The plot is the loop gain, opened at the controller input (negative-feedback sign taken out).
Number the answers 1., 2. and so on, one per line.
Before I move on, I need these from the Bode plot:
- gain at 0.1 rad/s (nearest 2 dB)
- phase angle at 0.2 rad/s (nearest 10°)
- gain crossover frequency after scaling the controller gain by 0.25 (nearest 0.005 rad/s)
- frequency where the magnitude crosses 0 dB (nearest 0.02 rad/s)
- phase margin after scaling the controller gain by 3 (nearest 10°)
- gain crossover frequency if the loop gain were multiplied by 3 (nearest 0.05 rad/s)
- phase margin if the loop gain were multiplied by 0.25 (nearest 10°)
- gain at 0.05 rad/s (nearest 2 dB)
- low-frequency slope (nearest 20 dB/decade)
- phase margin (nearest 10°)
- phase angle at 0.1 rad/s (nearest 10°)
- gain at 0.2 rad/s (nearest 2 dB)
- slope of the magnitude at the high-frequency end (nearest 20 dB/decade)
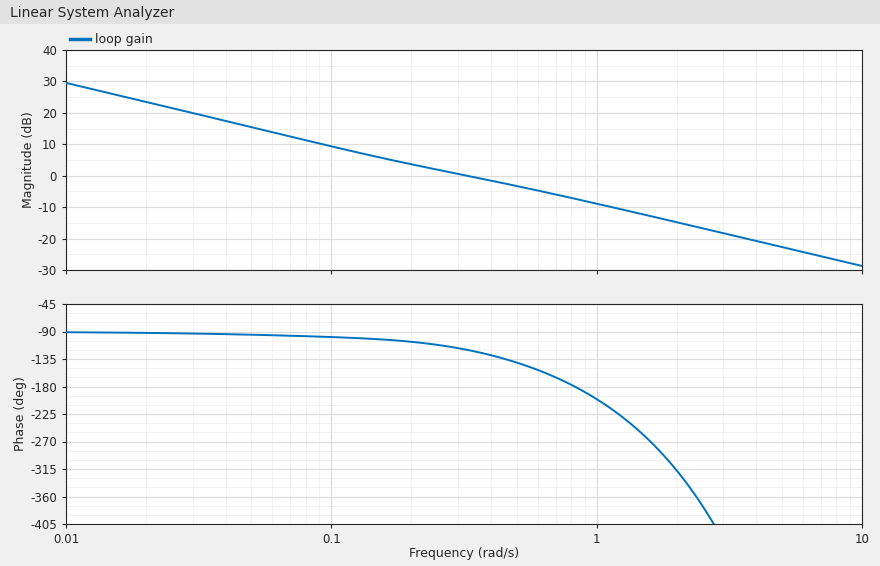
1. 10 dB
2. -110°
3. 0.075 rad/s
4. 0.32 rad/s
5. -30°
6. 1.10 rad/s
7. 80°
8. 16 dB
9. -20 dB/decade
10. 60°
11. -100°
12. 4 dB
13. -20 dB/decade
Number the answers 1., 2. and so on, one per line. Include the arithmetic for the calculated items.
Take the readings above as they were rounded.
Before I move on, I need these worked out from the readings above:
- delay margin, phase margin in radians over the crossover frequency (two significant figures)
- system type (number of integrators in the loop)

1. 60 × π / 180 / 0.32 = 3.3 s
2. 1
